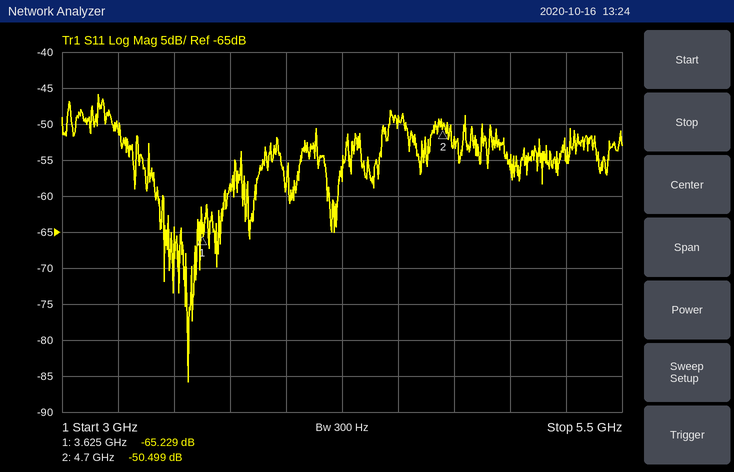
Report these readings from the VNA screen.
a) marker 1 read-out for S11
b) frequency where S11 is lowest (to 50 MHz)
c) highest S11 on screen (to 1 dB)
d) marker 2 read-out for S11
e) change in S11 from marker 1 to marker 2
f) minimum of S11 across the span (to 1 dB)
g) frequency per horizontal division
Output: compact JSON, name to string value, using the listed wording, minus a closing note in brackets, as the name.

{"marker 1 read-out for S11": "-65.229 dB", "frequency where S11 is lowest": "3.55 GHz", "highest S11 on screen": "-46 dB", "marker 2 read-out for S11": "-50.499 dB", "change in S11 from marker 1 to marker 2": "14.730 dB", "minimum of S11 across the span": "-86 dB", "frequency per horizontal division": "250 MHz"}
